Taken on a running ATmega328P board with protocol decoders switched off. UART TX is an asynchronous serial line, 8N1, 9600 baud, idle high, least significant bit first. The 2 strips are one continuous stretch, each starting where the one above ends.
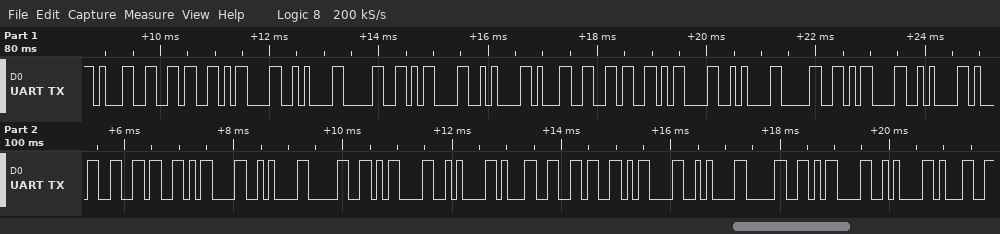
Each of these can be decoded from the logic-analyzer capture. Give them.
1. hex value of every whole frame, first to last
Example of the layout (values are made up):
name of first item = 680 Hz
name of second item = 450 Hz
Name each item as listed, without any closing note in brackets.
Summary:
hex value of every whole frame, first to last = 0x31 0x36 0x0D 0x0A 0x30 0x0D 0x0A 0x31 0x36 0x0D 0x0A 0x30 0x0D 0x0A 0x31 0x36 0x0D 0x0A 0x30 0x0D 0x0A 0x31 0x36 0x0D 0x0A 0x30 0x0D 0x0A 0x31
